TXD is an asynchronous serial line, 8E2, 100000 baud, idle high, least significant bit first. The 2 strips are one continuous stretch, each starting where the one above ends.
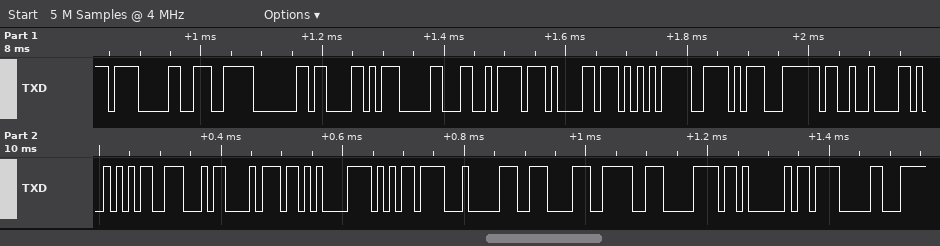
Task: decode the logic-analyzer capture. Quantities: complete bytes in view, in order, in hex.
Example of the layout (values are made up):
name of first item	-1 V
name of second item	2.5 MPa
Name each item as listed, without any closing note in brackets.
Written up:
complete bytes in view, in order, in hex	0x0F 0xCE 0xC0 0x58 0x30 0x7A 0x61 0xD5 0x5E 0xFC 0x12 0xA9 0x8E 0xE8 0x85 0xB5 0x04 0x0E 0x3E 0xF0 0x81 0x0F
